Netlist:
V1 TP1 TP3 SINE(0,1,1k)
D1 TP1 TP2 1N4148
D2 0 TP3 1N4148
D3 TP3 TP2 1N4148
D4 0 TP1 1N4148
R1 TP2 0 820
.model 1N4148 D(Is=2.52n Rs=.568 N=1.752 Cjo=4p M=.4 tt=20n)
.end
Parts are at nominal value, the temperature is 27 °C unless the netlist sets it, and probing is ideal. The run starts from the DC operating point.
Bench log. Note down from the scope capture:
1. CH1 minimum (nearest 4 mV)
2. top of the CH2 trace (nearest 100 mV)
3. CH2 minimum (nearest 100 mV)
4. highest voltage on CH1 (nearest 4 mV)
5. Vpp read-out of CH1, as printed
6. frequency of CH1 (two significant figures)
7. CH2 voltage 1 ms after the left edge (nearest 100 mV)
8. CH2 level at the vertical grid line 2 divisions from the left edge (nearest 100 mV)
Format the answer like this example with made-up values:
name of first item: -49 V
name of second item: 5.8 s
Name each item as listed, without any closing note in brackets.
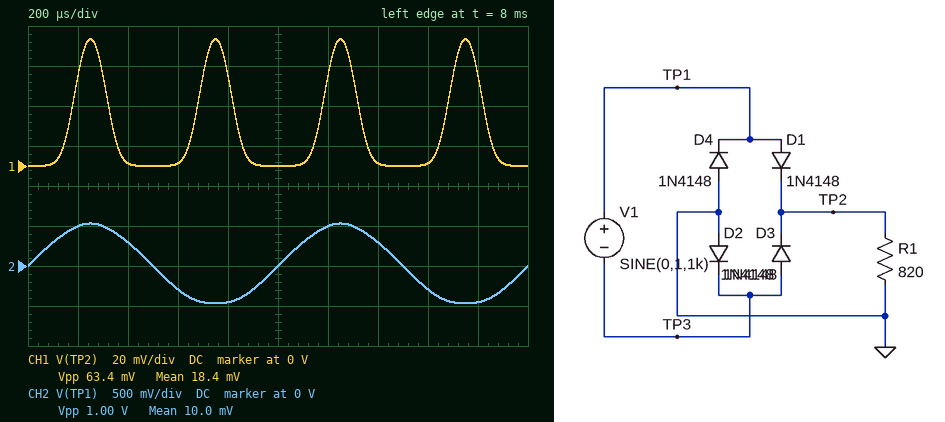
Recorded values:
CH1 minimum: 0 V
top of the CH2 trace: 500 mV
CH2 minimum: -500 mV
highest voltage on CH1: 64 mV
Vpp read-out of CH1, as printed: 63.4 mV
frequency of CH1: 2.0 kHz
CH2 voltage 1 ms after the left edge: 0 V
CH2 level at the vertical grid line 2 divisions from the left edge: 300 mV
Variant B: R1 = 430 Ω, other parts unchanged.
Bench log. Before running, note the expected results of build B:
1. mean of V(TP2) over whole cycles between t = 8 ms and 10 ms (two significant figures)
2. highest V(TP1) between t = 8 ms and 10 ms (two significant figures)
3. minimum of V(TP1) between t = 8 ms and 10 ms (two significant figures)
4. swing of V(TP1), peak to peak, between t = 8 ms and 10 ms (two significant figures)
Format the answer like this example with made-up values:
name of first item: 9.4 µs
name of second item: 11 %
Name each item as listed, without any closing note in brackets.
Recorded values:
mean of V(TP2) over whole cycles between t = 8 ms and 10 ms: 12 mV
highest V(TP1) between t = 8 ms and 10 ms: 520 mV
minimum of V(TP1) between t = 8 ms and 10 ms: -480 mV
swing of V(TP1), peak to peak, between t = 8 ms and 10 ms: 1.0 V
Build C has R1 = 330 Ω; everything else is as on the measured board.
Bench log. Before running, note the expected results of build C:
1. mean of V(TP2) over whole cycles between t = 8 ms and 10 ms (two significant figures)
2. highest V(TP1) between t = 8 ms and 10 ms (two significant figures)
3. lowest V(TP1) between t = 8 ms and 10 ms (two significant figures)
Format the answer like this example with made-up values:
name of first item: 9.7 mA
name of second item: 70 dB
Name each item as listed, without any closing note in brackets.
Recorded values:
mean of V(TP2) over whole cycles between t = 8 ms and 10 ms: 9.4 mV
highest V(TP1) between t = 8 ms and 10 ms: 520 mV
lowest V(TP1) between t = 8 ms and 10 ms: -480 mV
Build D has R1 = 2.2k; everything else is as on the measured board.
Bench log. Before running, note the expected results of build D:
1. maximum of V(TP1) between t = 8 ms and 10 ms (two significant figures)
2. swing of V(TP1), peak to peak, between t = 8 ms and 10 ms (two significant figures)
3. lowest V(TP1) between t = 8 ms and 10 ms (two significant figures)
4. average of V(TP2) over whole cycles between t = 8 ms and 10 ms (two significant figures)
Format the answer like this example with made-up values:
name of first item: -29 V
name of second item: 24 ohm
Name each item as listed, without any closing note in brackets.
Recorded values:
maximum of V(TP1) between t = 8 ms and 10 ms: 550 mV
swing of V(TP1), peak to peak, between t = 8 ms and 10 ms: 1.0 V
lowest V(TP1) between t = 8 ms and 10 ms: -450 mV
average of V(TP2) over whole cycles between t = 8 ms and 10 ms: 34 mV
